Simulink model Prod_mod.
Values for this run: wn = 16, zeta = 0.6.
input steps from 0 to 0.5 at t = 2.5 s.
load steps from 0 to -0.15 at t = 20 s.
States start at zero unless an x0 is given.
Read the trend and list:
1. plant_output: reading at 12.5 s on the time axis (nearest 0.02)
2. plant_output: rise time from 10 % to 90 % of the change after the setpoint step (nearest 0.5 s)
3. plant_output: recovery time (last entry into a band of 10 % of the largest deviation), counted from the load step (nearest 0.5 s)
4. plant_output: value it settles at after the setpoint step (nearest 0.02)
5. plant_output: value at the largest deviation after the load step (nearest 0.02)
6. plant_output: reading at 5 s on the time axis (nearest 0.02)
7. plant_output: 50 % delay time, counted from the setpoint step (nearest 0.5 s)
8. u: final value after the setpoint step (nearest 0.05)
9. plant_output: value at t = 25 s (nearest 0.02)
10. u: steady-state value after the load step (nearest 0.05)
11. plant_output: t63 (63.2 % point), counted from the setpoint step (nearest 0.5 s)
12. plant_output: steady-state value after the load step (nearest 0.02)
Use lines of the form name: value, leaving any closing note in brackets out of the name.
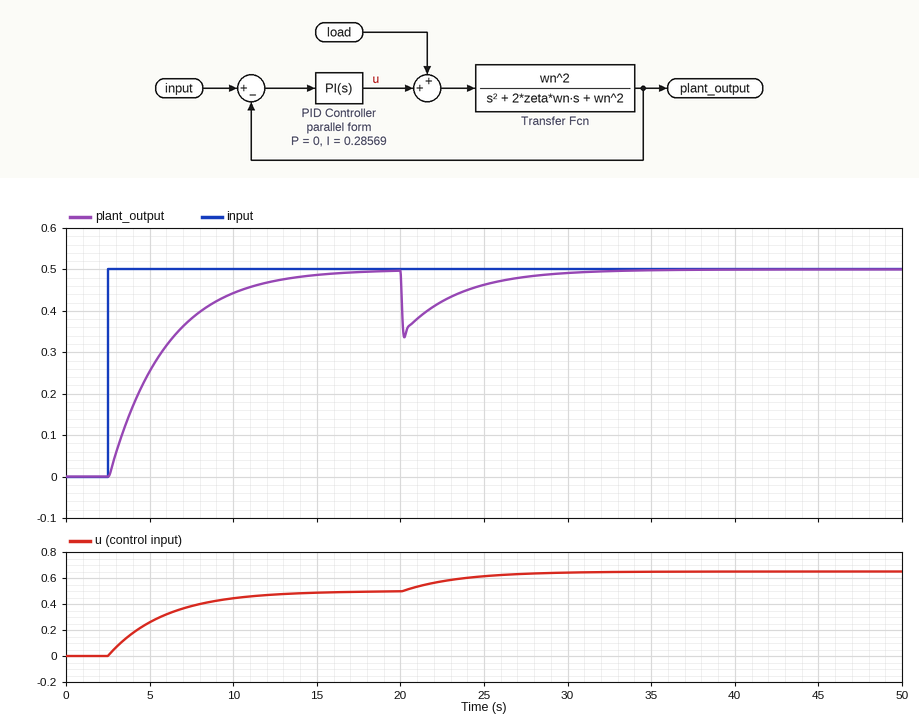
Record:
plant_output: reading at 12.5 s on the time axis: 0.48
plant_output: rise time from 10 % to 90 % of the change after the setpoint step: 7.5 s
plant_output: recovery time (last entry into a band of 10 % of the largest deviation), counted from the load step: 8.0 s
plant_output: value it settles at after the setpoint step: 0.50
plant_output: value at the largest deviation after the load step: 0.34
plant_output: reading at 5 s on the time axis: 0.26
plant_output: 50 % delay time, counted from the setpoint step: 2.5 s
u: final value after the setpoint step: 0.50
plant_output: value at t = 25 s: 0.46
u: steady-state value after the load step: 0.65
plant_output: t63 (63.2 % point), counted from the setpoint step: 3.5 s
plant_output: steady-state value after the load step: 0.50
